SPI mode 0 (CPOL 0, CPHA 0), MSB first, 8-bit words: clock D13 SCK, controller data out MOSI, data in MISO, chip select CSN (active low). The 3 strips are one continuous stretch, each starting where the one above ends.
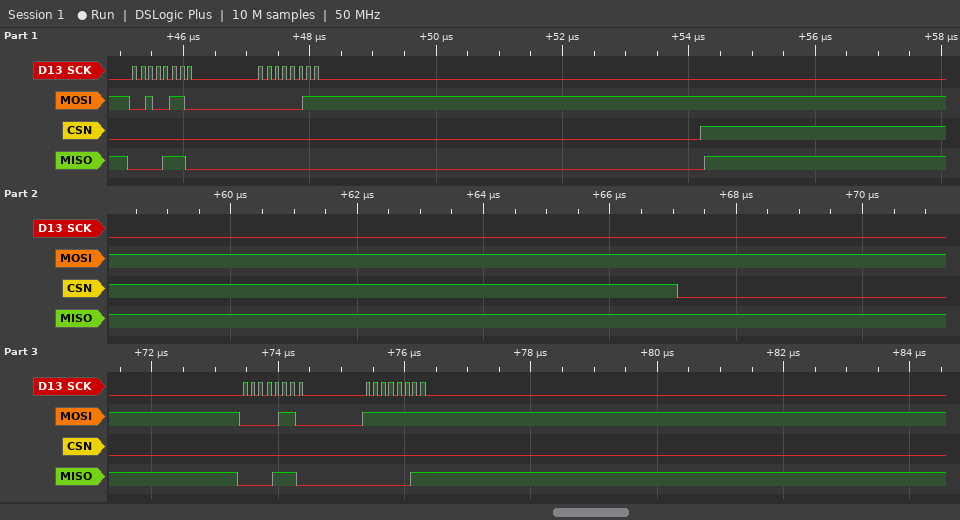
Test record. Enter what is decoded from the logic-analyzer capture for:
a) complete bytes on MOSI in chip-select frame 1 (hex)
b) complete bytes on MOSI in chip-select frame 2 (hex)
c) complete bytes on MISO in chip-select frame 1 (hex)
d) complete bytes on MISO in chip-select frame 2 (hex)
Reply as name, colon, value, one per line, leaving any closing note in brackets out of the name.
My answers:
complete bytes on MOSI in chip-select frame 1: 26 03
complete bytes on MOSI in chip-select frame 2: 06 FF
complete bytes on MISO in chip-select frame 1: 0E 00
complete bytes on MISO in chip-select frame 2: 0E 03
